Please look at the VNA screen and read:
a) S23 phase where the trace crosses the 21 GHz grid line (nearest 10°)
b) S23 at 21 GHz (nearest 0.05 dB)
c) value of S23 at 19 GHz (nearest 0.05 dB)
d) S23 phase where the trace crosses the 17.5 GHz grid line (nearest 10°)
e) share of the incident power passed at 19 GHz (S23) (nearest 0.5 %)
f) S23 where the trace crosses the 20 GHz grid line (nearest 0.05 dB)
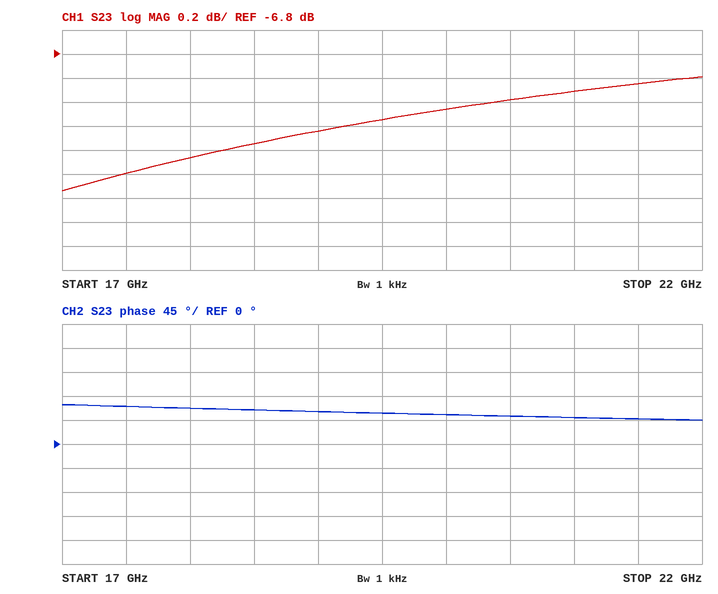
50°
-7.10 dB
-7.45 dB
70°
18.0 %
-7.25 dB
